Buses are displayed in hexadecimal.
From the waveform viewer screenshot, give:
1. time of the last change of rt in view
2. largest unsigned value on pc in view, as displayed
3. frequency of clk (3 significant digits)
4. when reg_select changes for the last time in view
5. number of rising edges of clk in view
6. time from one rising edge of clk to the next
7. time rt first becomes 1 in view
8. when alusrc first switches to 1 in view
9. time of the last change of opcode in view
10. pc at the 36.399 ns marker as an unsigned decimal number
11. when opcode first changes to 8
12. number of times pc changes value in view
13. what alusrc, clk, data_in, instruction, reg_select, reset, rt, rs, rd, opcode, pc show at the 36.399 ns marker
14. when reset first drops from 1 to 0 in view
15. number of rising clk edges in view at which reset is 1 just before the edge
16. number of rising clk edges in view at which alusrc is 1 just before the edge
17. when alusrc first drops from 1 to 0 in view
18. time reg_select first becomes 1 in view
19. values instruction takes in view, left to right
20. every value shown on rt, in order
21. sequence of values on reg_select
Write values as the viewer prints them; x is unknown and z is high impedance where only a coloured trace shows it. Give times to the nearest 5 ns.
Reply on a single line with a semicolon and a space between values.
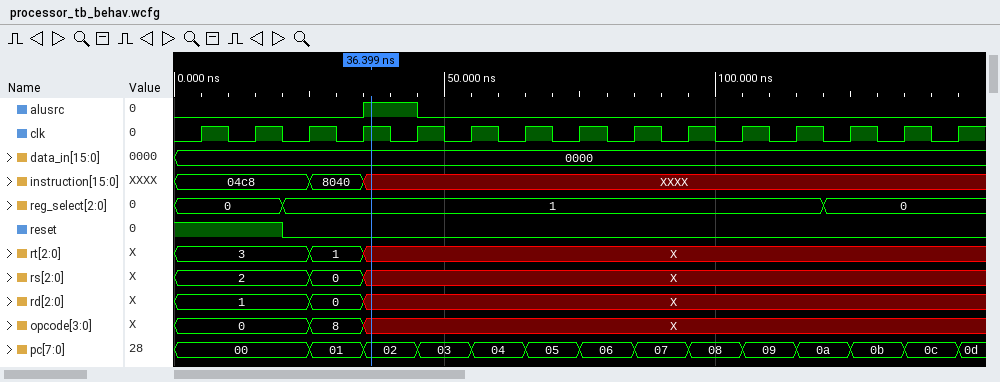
35 ns; 0d; 100 MHz; 120 ns; 15; 10 ns; 25 ns; 35 ns; 35 ns; 2; 25 ns; 13; alusrc=1, clk=1, data_in=0000, instruction=XXXX, reg_select=1, reset=0, rt=X, rs=X, rd=X, opcode=X, pc=02; 20 ns; 2; 1; 45 ns; 20 ns; 04c8, 8040, XXXX; 3, 1, X; 0, 1, 0
